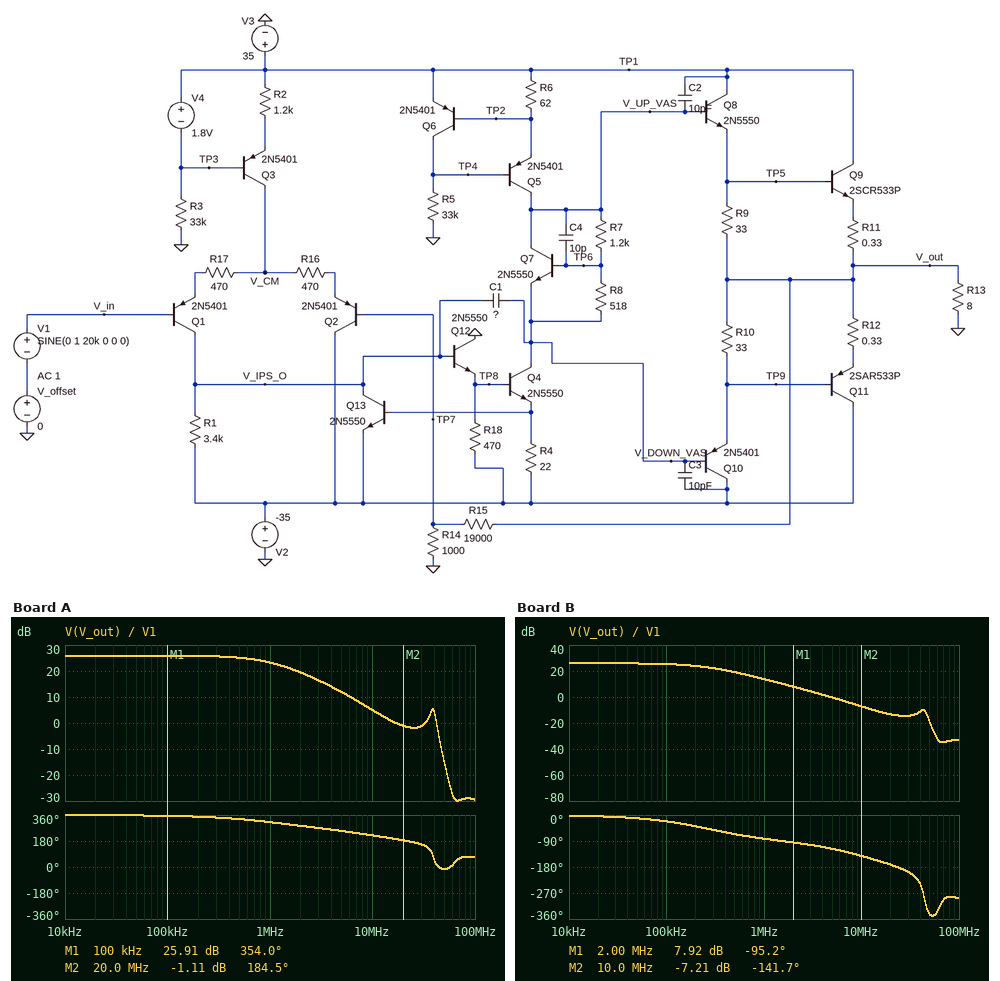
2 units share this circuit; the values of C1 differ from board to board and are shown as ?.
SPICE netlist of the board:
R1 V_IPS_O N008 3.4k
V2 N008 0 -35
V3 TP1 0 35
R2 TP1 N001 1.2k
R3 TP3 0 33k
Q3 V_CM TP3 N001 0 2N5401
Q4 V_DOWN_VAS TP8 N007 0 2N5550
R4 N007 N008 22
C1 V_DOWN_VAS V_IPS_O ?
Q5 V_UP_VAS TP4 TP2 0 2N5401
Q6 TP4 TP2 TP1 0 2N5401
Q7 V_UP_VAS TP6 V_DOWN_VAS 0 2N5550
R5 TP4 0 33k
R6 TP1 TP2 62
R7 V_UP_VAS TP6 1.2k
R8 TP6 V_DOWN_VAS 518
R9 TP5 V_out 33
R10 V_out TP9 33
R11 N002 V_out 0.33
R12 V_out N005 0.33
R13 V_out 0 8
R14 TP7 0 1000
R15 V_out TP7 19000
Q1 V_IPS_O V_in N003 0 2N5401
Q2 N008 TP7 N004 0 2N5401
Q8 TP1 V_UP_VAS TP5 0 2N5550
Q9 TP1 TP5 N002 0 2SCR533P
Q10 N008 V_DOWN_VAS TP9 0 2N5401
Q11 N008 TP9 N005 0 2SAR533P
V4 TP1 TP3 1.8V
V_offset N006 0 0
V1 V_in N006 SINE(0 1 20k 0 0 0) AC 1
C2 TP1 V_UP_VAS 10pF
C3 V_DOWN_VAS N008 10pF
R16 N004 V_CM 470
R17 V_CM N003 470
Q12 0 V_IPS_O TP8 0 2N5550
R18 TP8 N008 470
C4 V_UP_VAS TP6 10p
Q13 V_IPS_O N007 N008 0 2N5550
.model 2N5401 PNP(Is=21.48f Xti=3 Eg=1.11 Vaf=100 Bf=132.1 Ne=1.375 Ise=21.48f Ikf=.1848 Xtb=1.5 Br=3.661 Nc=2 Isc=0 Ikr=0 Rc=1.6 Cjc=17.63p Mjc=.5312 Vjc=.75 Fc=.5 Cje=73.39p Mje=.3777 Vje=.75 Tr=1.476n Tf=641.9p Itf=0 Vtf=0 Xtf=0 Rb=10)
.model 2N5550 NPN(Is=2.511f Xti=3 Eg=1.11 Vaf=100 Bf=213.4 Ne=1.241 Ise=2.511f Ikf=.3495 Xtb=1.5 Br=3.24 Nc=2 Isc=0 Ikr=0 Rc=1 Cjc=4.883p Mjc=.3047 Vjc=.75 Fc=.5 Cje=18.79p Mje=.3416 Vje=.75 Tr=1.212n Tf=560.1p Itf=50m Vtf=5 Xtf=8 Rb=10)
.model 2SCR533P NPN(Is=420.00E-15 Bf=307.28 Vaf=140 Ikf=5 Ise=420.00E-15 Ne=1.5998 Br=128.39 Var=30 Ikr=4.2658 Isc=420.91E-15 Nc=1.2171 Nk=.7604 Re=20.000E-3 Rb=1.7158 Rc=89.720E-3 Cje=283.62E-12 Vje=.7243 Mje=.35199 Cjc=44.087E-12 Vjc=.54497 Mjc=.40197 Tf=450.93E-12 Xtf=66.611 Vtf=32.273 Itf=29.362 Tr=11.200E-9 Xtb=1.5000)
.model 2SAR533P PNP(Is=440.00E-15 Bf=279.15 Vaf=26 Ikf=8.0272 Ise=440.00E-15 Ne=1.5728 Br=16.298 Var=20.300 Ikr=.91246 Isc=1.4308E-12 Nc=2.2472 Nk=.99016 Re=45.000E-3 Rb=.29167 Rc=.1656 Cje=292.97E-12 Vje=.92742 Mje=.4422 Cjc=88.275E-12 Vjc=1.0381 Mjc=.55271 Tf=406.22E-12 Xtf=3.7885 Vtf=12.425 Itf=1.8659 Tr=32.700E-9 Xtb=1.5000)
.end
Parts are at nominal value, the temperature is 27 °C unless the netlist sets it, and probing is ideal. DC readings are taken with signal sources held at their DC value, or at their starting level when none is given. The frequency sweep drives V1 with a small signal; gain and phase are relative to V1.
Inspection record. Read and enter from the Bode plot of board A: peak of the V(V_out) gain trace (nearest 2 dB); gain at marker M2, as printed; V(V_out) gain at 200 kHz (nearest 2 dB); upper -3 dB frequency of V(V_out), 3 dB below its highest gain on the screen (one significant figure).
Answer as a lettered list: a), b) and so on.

a) 26 dB
b) -1.11 dB
c) 26 dB
d) 1 MHz
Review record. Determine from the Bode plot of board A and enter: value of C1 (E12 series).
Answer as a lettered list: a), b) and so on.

a) 6.8 pF
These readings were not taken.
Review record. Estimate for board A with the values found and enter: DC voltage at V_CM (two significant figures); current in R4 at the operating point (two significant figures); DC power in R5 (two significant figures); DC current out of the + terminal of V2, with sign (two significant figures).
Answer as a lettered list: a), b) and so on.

a) 850 mV
b) 10 mA
c) 34 mW
d) -26 mA
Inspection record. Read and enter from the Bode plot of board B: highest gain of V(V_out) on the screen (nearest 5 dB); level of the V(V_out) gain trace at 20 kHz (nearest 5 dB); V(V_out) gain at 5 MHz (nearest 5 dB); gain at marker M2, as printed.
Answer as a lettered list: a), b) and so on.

a) 25 dB
b) 25 dB
c) 0 dB
d) -7.21 dB
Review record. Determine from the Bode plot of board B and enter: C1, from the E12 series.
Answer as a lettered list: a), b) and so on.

a) 27 pF
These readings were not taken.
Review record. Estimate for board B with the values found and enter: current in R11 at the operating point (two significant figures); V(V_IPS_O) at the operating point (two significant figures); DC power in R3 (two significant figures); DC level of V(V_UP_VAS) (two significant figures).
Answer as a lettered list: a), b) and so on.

a) 53 mA
b) -33 V
c) 33 mW
d) 1.9 V
